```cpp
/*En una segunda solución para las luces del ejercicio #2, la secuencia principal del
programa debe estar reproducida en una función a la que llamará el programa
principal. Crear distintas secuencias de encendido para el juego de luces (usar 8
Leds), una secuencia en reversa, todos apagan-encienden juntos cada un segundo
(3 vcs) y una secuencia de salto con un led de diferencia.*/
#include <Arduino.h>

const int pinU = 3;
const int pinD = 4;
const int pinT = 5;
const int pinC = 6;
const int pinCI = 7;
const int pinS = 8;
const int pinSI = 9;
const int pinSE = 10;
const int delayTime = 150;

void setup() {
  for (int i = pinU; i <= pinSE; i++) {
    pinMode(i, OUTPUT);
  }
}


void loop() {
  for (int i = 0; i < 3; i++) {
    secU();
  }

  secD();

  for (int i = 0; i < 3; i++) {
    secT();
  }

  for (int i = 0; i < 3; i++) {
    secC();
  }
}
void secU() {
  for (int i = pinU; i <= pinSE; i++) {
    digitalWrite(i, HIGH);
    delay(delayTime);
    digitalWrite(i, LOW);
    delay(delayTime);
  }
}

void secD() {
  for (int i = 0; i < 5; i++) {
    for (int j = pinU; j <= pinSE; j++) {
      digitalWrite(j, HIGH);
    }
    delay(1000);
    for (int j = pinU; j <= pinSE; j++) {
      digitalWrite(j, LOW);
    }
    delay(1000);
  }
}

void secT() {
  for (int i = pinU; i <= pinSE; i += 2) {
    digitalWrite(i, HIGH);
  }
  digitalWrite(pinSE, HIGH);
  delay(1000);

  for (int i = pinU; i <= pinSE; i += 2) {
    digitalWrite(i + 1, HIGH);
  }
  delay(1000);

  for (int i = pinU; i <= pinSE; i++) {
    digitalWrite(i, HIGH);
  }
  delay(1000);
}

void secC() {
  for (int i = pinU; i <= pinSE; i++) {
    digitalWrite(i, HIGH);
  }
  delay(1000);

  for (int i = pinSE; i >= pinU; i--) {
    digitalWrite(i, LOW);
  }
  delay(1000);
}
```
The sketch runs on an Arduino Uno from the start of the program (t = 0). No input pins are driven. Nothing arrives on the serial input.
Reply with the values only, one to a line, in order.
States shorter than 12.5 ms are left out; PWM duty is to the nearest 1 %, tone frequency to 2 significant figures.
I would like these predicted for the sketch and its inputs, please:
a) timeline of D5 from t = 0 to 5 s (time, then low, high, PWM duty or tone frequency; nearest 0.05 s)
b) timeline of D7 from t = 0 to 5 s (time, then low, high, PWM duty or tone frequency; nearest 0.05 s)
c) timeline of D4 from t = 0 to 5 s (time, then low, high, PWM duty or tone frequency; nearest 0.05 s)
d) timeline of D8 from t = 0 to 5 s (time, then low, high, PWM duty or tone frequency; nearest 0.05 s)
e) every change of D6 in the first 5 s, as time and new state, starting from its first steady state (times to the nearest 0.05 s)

0 s low; 0.6 s high; 0.75 s low; 3 s high; 3.15 s low
0 s low; 1.2 s high; 1.35 s low; 3.6 s high; 3.75 s low
0 s low; 0.3 s high; 0.45 s low; 2.7 s high; 2.85 s low
0 s low; 1.5 s high; 1.65 s low; 3.9 s high; 4.05 s low
0 s low; 0.9 s high; 1.05 s low; 3.3 s high; 3.45 s low
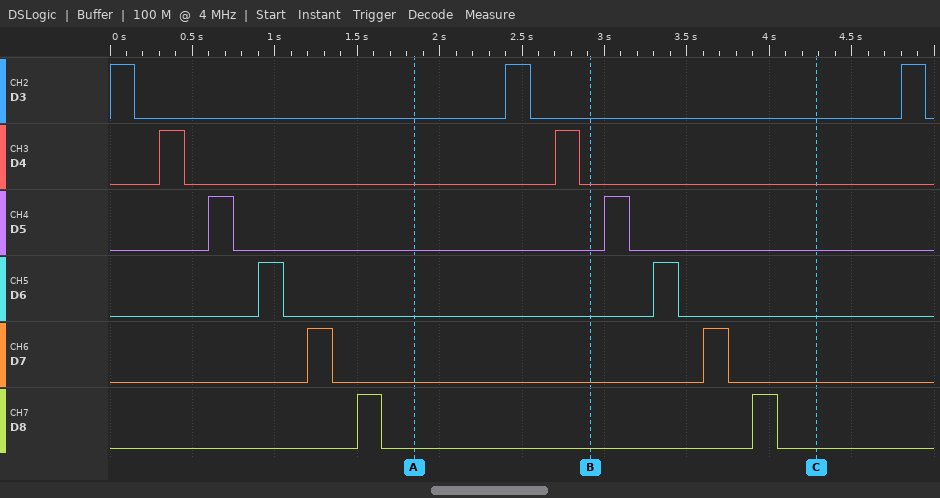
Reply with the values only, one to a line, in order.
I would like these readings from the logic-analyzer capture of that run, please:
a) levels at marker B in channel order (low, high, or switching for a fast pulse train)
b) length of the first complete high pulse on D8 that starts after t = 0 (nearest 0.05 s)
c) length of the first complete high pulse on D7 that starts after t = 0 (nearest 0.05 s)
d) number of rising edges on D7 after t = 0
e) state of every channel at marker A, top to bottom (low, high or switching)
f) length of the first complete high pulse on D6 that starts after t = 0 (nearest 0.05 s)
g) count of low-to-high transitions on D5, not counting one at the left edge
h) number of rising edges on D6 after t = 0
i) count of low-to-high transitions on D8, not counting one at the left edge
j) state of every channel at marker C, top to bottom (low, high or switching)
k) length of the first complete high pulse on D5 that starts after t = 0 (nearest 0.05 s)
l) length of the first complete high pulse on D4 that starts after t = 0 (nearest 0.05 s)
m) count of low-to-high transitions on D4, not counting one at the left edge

D3 low, D4 low, D5 low, D6 low, D7 low, D8 low
0.15 s
0.15 s
2
D3 low, D4 low, D5 low, D6 low, D7 low, D8 low
0.15 s
2
2
2
D3 low, D4 low, D5 low, D6 low, D7 low, D8 low
0.15 s
0.15 s
2
